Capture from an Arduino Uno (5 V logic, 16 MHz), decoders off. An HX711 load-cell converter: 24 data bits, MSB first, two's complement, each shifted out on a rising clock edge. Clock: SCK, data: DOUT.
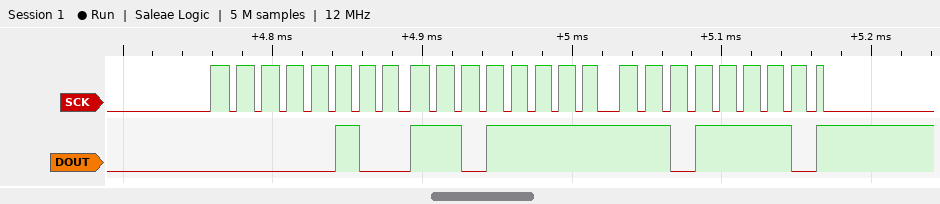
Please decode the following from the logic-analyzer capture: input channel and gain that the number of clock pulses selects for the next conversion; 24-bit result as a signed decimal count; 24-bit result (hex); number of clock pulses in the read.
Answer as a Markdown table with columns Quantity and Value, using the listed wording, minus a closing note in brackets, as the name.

| Quantity | Value |
|---|---|
| input channel and gain that the number of clock pulses selects for the next conversion | channel A, gain 128 |
| 24-bit result as a signed decimal count | 319454 |
| 24-bit result | 0x04DFDE |
| number of clock pulses in the read | 25 |
